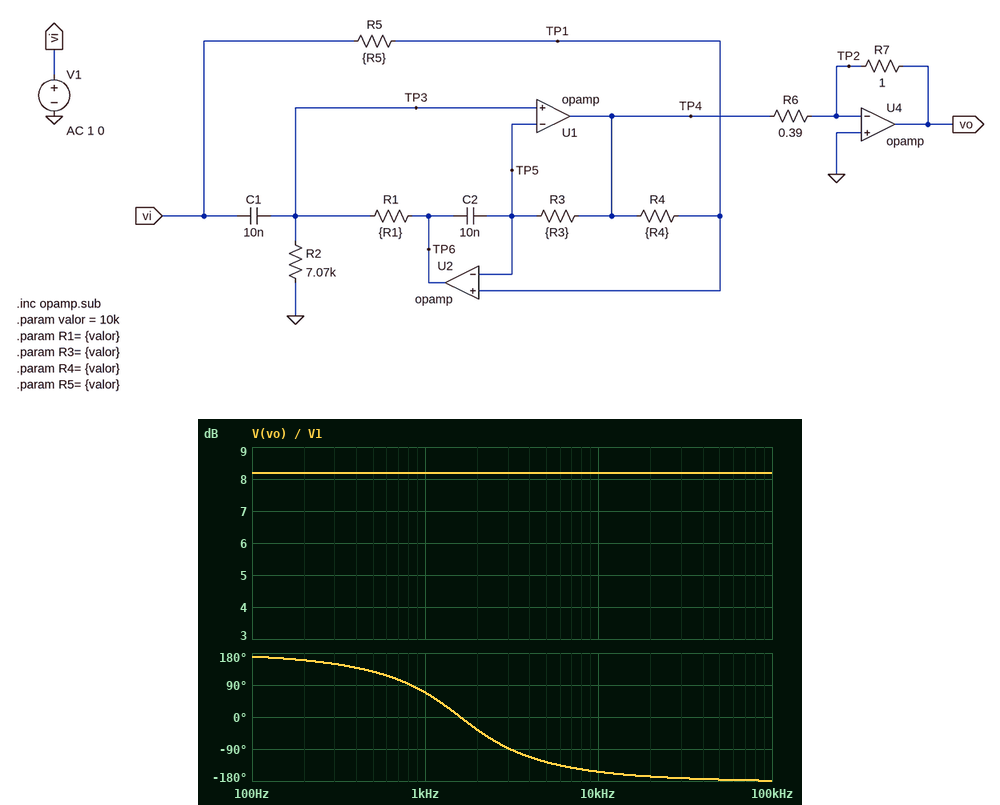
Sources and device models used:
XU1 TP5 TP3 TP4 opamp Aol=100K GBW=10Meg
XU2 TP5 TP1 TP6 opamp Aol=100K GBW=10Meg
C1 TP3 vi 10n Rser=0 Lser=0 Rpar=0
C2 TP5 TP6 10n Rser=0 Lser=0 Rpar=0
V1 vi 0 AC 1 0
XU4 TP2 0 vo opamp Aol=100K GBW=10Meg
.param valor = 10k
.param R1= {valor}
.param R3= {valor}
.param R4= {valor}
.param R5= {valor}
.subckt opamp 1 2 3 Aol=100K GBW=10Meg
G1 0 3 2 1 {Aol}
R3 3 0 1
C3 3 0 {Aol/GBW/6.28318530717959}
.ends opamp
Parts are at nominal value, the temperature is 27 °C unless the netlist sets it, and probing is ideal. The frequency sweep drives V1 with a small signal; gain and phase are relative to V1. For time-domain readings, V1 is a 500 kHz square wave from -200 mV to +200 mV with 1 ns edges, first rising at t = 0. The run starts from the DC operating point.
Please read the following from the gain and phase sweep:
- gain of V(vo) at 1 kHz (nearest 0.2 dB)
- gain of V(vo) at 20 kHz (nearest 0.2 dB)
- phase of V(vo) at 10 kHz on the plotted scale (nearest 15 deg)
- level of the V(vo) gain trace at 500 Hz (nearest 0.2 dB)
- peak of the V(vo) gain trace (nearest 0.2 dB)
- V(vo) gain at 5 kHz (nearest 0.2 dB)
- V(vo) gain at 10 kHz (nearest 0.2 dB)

8.2 dB
8.2 dB
-150 deg
8.2 dB
8.2 dB
8.2 dB
8.2 dB
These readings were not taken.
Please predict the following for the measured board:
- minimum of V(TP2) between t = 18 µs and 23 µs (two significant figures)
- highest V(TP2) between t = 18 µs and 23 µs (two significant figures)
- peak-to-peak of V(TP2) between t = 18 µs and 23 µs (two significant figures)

-230 mV
230 mV
460 mV
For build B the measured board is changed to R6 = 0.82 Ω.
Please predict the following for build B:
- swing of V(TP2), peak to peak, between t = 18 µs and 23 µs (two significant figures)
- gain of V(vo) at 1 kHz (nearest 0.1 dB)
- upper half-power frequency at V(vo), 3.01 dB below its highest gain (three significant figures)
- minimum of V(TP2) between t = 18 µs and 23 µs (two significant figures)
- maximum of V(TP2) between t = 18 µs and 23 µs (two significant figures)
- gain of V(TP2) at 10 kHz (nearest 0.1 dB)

300 mV
1.7 dB
6.57 MHz
-150 mV
150 mV
-58.3 dB
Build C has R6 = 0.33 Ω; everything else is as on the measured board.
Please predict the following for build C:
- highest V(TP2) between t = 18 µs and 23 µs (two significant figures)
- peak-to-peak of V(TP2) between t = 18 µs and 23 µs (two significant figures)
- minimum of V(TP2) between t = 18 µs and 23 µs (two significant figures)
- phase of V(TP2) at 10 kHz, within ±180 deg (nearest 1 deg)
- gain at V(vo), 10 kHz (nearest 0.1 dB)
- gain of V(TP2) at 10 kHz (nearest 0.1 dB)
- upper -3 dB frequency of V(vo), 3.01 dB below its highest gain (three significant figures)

250 mV
500 mV
-250 mV
115 deg
9.6 dB
-50.4 dB
3.26 MHz
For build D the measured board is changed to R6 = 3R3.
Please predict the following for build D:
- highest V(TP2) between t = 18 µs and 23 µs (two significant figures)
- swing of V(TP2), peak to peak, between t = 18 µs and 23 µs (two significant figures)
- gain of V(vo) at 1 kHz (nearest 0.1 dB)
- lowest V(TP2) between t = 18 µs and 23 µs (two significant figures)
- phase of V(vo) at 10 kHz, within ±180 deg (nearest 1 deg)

50 mV
99 mV
-10.4 dB
-50 mV
-154 deg
